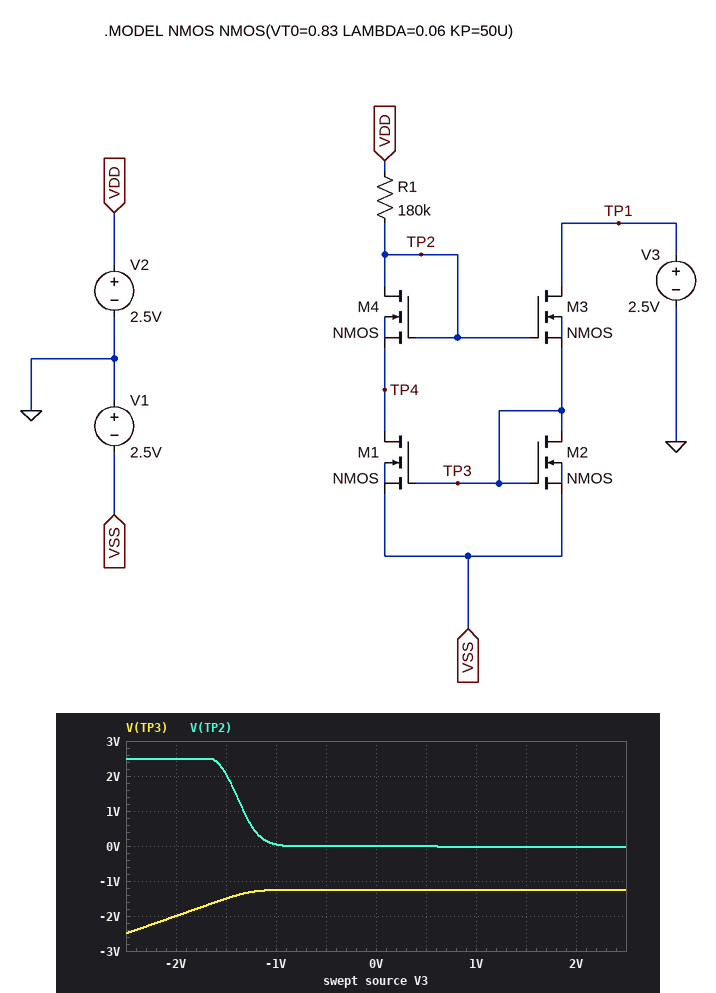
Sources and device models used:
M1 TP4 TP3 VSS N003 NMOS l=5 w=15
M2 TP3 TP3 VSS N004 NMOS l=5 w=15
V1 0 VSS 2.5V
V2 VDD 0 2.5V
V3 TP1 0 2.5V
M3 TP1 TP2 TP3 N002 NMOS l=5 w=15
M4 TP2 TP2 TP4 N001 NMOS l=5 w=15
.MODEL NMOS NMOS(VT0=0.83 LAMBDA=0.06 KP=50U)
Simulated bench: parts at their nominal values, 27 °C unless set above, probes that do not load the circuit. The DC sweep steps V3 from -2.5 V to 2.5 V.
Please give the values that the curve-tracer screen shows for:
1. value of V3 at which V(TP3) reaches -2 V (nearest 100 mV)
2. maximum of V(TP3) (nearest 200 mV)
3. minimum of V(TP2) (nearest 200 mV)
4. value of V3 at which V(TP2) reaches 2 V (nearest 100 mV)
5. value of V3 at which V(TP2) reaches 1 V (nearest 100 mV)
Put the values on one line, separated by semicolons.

-2.0 V; -1.2 V; 0 V; -1.5 V; -1.3 V
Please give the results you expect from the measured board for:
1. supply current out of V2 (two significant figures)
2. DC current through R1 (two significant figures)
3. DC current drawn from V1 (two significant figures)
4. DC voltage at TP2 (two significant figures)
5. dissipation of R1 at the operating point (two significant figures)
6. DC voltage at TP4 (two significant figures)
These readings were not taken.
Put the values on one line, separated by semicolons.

14 µA; 14 µA; 28 µA; -31 mV; 36 µW; -1.3 V
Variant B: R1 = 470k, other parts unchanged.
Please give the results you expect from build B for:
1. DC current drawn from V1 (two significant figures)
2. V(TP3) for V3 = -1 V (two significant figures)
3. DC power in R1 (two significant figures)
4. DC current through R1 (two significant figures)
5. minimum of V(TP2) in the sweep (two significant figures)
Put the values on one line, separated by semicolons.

12 µA; -1.4 V; 17 µW; 6.0 µA; -310 mV
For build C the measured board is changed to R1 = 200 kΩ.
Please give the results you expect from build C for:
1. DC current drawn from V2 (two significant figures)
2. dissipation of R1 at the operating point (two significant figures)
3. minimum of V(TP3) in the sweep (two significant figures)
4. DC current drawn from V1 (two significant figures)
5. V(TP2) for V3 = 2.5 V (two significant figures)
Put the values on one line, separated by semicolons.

13 µA; 33 µW; -2.5 V; 26 µA; -67 mV
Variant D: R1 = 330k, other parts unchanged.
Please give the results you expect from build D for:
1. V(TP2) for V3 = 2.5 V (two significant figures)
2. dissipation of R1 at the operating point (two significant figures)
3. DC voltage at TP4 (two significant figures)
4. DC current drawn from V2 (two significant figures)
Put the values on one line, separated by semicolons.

-220 mV; 22 µW; -1.4 V; 8.2 µA
